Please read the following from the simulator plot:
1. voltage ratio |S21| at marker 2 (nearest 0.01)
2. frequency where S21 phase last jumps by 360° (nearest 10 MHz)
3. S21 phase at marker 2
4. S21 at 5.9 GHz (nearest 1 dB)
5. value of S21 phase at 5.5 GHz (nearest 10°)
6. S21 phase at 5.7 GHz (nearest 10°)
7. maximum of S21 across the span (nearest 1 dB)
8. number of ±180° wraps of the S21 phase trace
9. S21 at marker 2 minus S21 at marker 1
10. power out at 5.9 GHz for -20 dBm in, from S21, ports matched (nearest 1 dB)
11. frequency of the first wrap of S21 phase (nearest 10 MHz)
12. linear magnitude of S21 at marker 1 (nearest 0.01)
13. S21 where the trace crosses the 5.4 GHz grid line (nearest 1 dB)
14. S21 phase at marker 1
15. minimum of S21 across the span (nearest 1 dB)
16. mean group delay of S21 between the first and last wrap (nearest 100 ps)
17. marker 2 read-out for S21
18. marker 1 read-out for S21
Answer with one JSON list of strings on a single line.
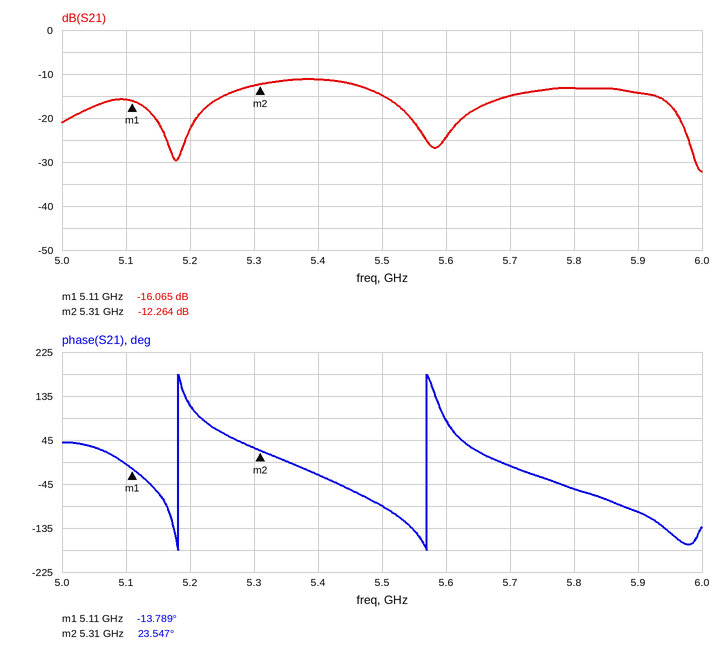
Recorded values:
["0.24", "5.57 GHz", "23.547°", "-14 dB", "-90°", "-10°", "-11 dB", "2", "3.801 dB", "-34 dBm", "5.18 GHz", "0.16", "-11 dB", "-13.789°", "-32 dB", "2.6 ns", "-12.264 dB", "-16.065 dB"]
